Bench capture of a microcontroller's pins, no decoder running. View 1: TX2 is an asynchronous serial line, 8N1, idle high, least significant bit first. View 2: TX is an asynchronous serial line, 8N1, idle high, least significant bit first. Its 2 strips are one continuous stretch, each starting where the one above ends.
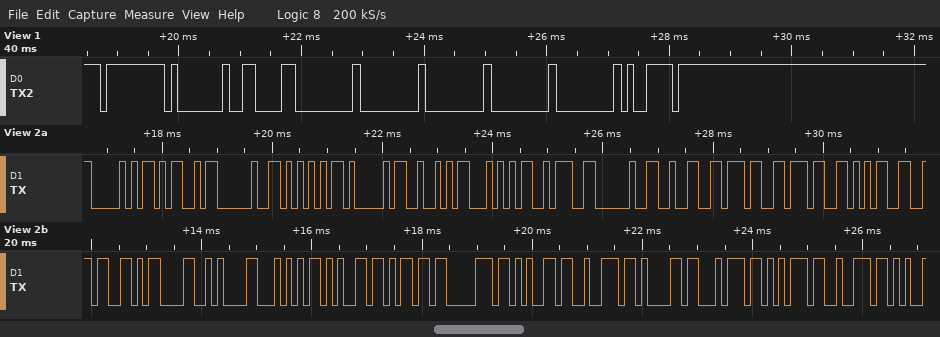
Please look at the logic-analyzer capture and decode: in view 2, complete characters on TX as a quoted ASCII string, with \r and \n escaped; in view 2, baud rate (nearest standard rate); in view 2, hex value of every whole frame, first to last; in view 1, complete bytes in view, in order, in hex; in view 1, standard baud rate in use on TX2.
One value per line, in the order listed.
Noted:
"PM UART: 27756\r\nTemperatur"
9600 baud
50 4D 20 55 41 52 54 3A 20 32 37 37 35 36 0D 0A 54 65 6D 70 65 72 61 74 75 72
FF 01 86 00 00 00 00 00 79
9600 baud
